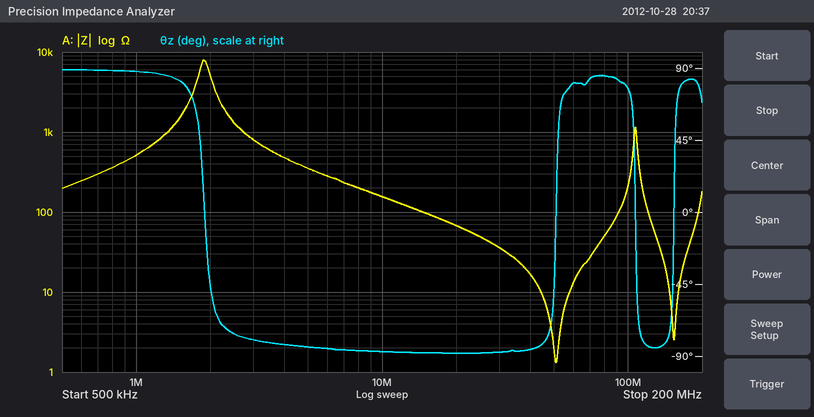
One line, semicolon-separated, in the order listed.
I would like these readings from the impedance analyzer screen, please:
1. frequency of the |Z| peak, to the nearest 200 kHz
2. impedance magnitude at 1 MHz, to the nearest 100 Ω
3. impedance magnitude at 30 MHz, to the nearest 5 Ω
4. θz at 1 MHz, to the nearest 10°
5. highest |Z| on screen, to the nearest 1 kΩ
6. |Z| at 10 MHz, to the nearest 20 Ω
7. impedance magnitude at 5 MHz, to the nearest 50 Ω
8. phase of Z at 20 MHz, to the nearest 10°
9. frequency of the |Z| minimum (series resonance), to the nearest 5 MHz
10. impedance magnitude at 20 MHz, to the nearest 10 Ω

1.8 MHz; 500 Ω; 35 Ω; 90°; 8 kΩ; 160 Ω; 350 Ω; -90°; 50 MHz; 70 Ω
